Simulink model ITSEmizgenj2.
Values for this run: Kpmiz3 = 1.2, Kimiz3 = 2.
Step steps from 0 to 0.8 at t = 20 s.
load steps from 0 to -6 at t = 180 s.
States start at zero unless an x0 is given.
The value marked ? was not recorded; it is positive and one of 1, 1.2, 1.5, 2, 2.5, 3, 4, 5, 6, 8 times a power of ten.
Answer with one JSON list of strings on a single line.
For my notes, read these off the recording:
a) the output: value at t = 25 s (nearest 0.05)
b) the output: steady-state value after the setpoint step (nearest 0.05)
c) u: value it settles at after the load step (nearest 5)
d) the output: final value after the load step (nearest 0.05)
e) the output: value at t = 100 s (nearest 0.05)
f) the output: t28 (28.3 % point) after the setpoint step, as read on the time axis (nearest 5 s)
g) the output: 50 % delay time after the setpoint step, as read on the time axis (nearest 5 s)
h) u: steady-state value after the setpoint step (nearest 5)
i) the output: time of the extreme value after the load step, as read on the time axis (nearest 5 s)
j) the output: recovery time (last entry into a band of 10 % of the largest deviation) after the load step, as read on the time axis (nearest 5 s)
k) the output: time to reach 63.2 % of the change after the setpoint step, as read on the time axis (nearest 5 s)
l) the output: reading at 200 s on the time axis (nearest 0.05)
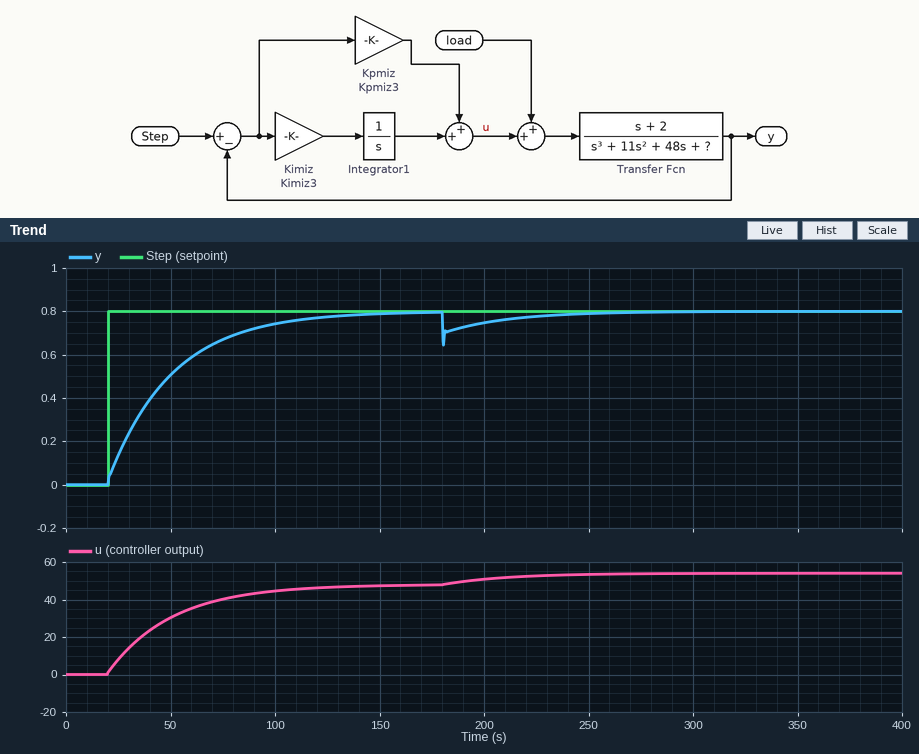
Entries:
["0.15", "0.80", "55", "0.80", "0.75", "30 s", "40 s", "50", "180 s", "240 s", "50 s", "0.75"]
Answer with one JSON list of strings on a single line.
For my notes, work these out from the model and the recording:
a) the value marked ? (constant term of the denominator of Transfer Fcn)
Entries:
["120"]
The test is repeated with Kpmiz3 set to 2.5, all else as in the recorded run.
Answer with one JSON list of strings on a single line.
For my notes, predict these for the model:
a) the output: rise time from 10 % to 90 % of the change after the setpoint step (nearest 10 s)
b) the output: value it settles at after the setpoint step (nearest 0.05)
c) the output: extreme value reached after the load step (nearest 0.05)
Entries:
["70 s", "0.80", "0.65"]
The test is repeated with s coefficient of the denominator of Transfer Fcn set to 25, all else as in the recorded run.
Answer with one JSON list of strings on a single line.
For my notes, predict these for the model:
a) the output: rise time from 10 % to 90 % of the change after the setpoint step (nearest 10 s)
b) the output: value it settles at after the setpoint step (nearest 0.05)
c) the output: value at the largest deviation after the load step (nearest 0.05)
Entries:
["70 s", "0.80", "0.60"]
